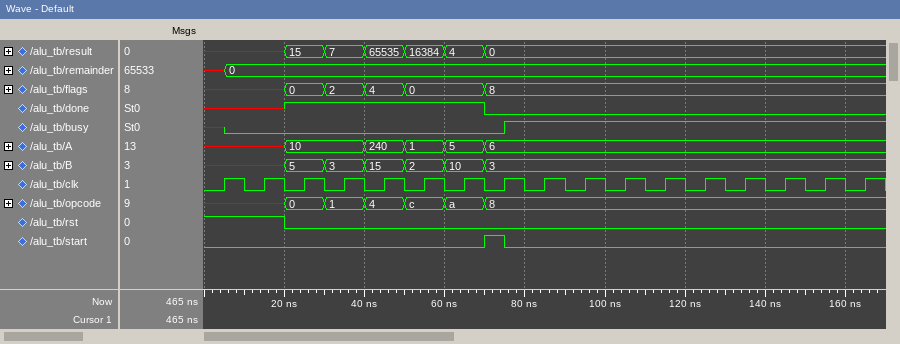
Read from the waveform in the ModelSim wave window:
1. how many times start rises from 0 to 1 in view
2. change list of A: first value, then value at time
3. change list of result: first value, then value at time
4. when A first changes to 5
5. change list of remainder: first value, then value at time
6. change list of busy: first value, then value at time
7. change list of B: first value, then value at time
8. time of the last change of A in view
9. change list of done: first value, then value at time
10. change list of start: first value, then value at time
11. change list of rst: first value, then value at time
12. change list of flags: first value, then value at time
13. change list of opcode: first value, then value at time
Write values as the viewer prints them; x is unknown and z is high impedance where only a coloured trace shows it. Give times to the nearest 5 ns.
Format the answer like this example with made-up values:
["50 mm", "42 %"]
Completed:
["1", "x, 10 at 20 ns, 240 at 40 ns, 1 at 50 ns, 5 at 60 ns, 6 at 70 ns", "x, 15 at 20 ns, 7 at 30 ns, 65535 at 40 ns, 16384 at 50 ns, 4 at 60 ns, 0 at 70 ns", "60 ns", "x, 0 at 5 ns", "x, 0 at 5 ns, 1 at 75 ns", "x, 5 at 20 ns, 3 at 30 ns, 15 at 40 ns, 2 at 50 ns, 10 at 60 ns, 3 at 70 ns", "70 ns", "x, 1 at 20 ns, 0 at 70 ns", "0, 1 at 70 ns, 0 at 75 ns", "1, 0 at 20 ns", "x, 0 at 20 ns, 2 at 30 ns, 4 at 40 ns, 0 at 50 ns, 8 at 70 ns", "x, 0 at 20 ns, 1 at 30 ns, 4 at 40 ns, c at 50 ns, a at 60 ns, 8 at 70 ns"]
